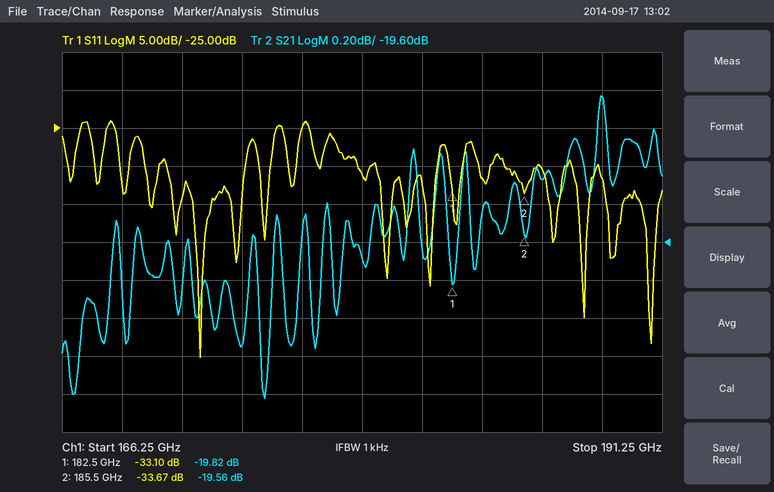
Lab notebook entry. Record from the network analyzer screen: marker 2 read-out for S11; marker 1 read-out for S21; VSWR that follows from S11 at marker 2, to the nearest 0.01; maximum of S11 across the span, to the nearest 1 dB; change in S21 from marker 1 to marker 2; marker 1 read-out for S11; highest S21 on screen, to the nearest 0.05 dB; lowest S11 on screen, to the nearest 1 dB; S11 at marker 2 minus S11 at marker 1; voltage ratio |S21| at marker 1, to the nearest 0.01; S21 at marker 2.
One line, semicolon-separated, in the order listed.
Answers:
-33.67 dB; -19.82 dB; 1.04; -24 dB; 0.26 dB; -33.10 dB; -18.85 dB; -55 dB; -0.57 dB; 0.10; -19.56 dB
